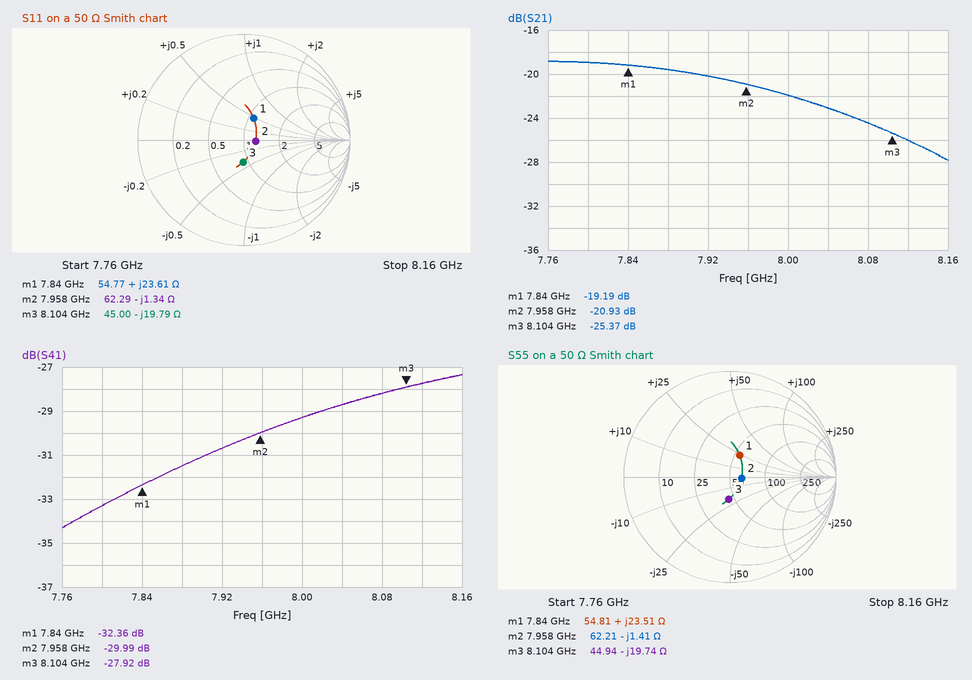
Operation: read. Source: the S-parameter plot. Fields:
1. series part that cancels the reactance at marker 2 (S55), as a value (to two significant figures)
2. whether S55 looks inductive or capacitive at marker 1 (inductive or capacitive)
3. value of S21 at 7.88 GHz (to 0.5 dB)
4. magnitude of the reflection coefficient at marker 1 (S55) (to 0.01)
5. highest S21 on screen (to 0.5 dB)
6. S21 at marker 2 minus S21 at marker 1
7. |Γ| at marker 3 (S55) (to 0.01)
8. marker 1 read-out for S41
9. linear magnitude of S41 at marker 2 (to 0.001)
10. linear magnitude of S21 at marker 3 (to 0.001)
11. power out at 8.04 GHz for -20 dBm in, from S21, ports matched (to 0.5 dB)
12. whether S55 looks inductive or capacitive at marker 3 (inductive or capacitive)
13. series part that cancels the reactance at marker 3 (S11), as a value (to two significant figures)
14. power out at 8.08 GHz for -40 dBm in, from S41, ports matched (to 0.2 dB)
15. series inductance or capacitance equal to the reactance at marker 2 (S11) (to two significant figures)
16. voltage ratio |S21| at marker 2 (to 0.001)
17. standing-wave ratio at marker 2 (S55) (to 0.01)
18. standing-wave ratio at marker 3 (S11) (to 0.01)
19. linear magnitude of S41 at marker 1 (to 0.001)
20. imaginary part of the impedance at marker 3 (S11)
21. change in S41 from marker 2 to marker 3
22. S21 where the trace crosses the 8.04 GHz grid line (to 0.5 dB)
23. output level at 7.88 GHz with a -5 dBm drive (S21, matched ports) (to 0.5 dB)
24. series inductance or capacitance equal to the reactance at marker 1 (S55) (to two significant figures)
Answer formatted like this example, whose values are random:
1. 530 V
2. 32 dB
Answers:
1. 28 pH
2. inductive
3. -19.5 dB
4. 0.22
5. -19.0 dB
6. -1.74 dB
7. 0.21
8. -32.36 dB
9. 0.032
10. 0.054
11. -43.0 dBm
12. capacitive
13. 390 pH
14. -68.2 dBm
15. 15 pF
16. 0.090
17. 1.25
18. 1.53
19. 0.024
20. -19.79 Ω
21. 2.07 dB
22. -23.0 dB
23. -24.5 dBm
24. 480 pH
